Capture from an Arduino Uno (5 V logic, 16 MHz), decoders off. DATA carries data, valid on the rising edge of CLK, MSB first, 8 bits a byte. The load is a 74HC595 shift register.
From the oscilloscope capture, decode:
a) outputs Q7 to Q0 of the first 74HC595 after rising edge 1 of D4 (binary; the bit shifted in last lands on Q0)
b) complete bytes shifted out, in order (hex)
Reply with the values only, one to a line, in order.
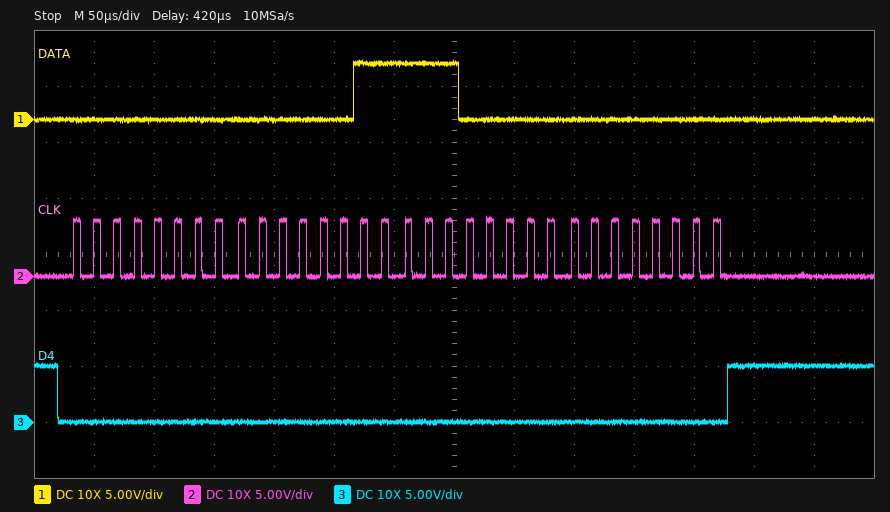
00000000
00 03 E0 00
